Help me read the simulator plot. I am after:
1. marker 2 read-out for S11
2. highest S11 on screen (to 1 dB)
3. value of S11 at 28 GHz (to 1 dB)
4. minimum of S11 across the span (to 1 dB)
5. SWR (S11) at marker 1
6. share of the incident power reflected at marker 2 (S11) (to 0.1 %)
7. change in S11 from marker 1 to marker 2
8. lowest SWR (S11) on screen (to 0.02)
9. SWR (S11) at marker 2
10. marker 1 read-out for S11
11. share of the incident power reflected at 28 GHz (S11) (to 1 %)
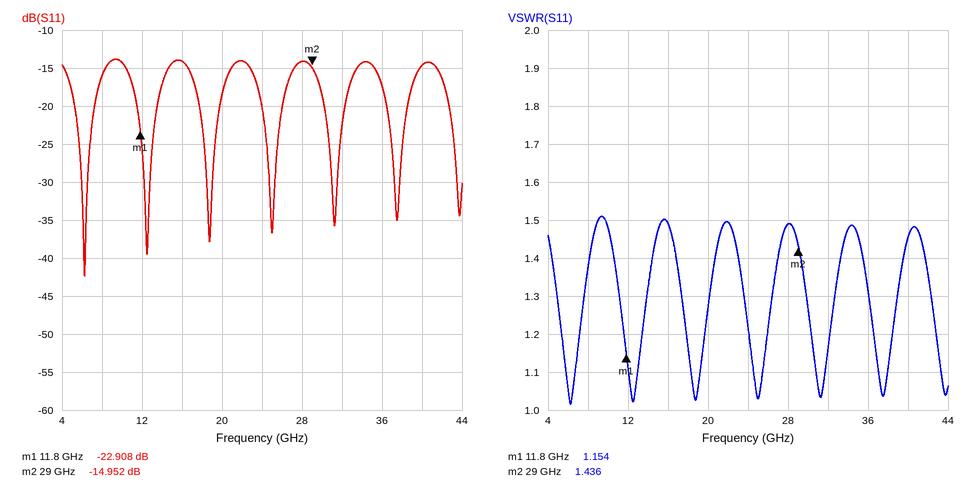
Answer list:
-14.952 dB
-14 dB
-14 dB
-42 dB
1.154
3.2 %
7.956 dB
1.02
1.436
-22.908 dB
4 %
